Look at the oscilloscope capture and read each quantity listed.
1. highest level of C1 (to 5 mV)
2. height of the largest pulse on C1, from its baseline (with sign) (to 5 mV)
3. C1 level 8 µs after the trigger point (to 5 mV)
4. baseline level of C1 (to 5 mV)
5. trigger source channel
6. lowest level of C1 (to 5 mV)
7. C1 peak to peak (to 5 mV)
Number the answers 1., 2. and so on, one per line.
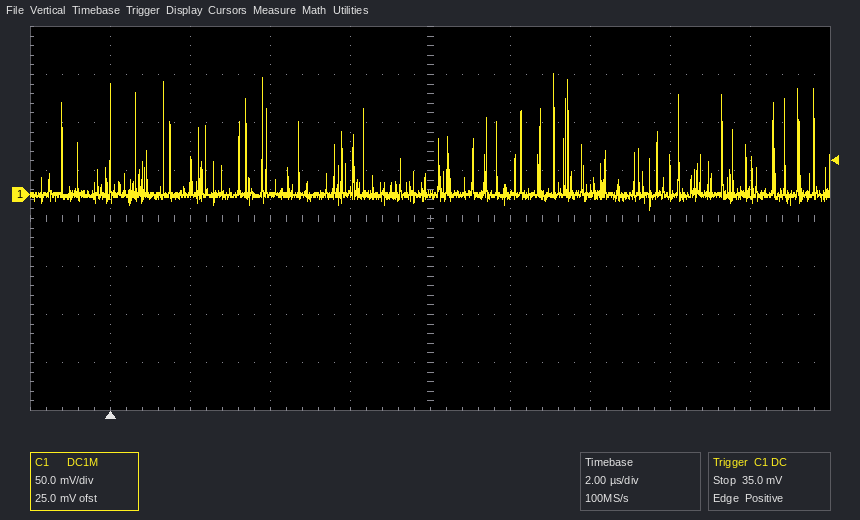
1. 125 mV
2. +125 mV
3. 0 mV
4. 0 mV
5. C1
6. -15 mV
7. 140 mV
